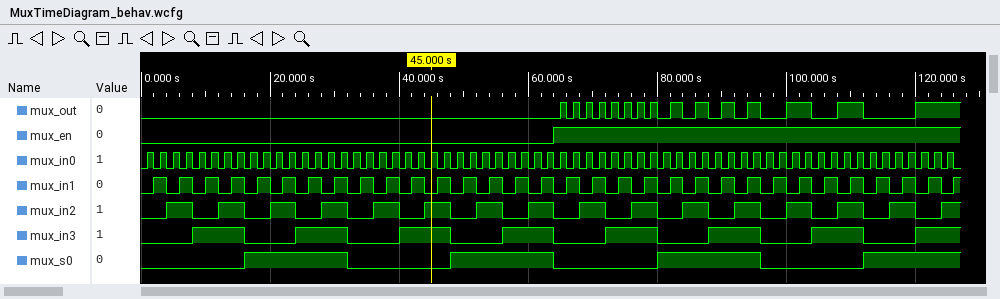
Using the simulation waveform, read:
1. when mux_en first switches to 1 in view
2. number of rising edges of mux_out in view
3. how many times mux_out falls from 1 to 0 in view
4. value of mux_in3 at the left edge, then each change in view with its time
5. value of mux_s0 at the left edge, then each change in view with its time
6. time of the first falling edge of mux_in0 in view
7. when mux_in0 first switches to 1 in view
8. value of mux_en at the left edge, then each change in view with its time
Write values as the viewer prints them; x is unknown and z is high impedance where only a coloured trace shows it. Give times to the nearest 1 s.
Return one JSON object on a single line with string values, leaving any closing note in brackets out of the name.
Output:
{"when mux_en first switches to 1 in view": "64 s", "number of rising edges of mux_out in view": "15", "how many times mux_out falls from 1 to 0 in view": "14", "value of mux_in3 at the left edge, then each change in view with its time": "0, 1 at 8 s, 0 at 16 s, 1 at 24 s, 0 at 32 s, 1 at 40 s, 0 at 48 s, 1 at 56 s, 0 at 64 s, 1 at 72 s, 0 at 80 s, 1 at 88 s, 0 at 96 s, 1 at 104 s, 0 at 112 s, 1 at 120 s", "value of mux_s0 at the left edge, then each change in view with its time": "0, 1 at 16 s, 0 at 32 s, 1 at 48 s, 0 at 64 s, 1 at 80 s, 0 at 96 s, 1 at 112 s", "time of the first falling edge of mux_in0 in view": "2 s", "when mux_in0 first switches to 1 in view": "1 s", "value of mux_en at the left edge, then each change in view with its time": "0, 1 at 64 s"}
